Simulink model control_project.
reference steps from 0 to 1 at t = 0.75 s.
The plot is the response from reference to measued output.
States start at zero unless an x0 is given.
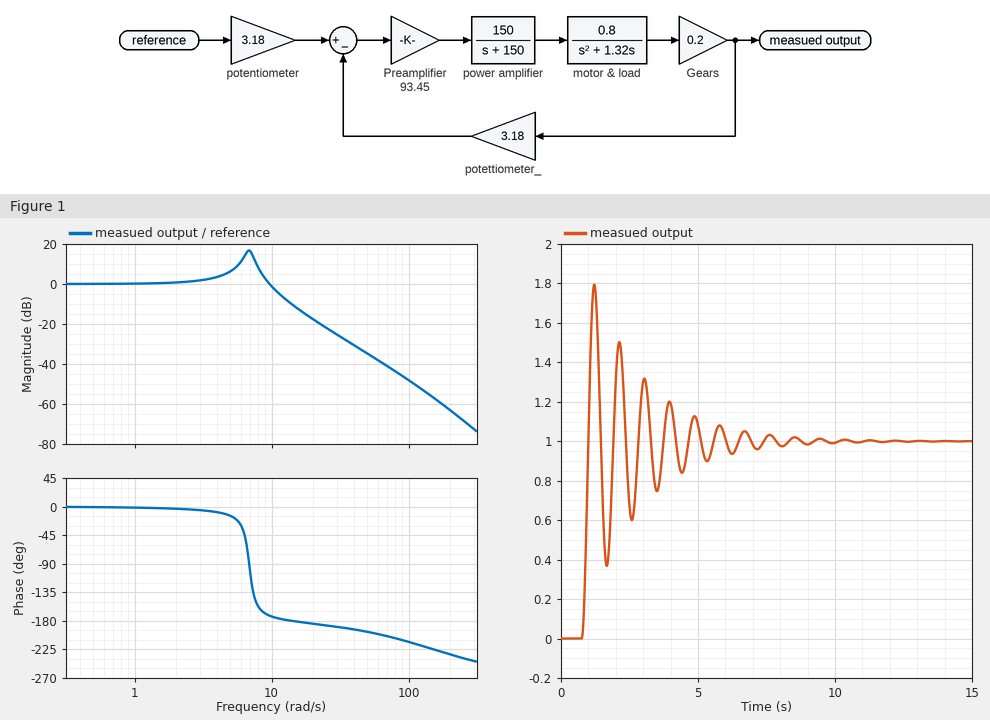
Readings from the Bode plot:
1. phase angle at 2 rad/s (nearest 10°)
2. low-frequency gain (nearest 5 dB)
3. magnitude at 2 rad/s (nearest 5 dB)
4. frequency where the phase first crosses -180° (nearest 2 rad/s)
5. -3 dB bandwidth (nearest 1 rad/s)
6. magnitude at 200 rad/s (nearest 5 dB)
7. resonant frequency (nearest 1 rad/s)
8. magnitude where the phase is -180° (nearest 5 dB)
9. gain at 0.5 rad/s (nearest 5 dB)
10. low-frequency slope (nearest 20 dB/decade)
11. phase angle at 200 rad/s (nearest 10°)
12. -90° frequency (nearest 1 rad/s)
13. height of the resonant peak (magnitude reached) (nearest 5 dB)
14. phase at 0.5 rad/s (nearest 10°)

0°
0 dB
0 dB
14 rad/s
11 rad/s
-65 dB
7 rad/s
-10 dB
0 dB
0 dB/decade
-230°
7 rad/s
15 dB
0°
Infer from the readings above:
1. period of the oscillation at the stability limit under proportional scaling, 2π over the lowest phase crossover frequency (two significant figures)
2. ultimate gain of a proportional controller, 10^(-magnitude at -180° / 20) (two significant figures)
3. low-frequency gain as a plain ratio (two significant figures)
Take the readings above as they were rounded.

0.45 s
3.2
1.0
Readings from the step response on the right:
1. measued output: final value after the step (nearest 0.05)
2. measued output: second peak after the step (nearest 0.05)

1.00
1.50
